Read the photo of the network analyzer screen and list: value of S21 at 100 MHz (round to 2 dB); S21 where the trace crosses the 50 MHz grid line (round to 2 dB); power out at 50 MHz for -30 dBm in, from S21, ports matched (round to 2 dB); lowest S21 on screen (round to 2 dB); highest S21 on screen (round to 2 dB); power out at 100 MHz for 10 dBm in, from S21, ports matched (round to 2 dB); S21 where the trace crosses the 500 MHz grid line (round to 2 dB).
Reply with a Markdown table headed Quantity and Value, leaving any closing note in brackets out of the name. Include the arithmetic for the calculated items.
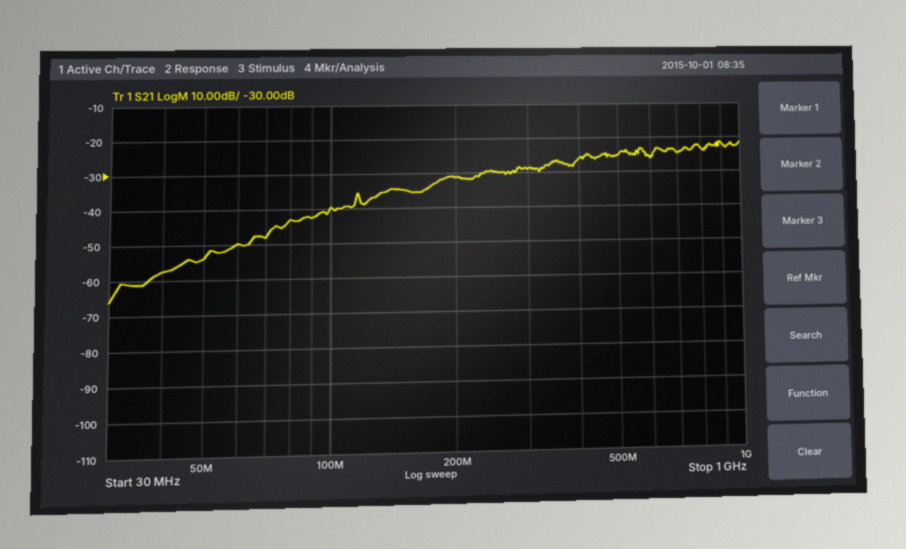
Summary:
| Quantity | Value |
|---|---|
| value of S21 at 100 MHz | -40 dB |
| S21 where the trace crosses the 50 MHz grid line | -54 dB |
| power out at 50 MHz for -30 dBm in, from S21, ports matched | -30 dBm + (-54 dB) = -84 dBm |
| lowest S21 on screen | -66 dB |
| highest S21 on screen | -22 dB |
| power out at 100 MHz for 10 dBm in, from S21, ports matched | 10 dBm + (-40 dB) = -30 dBm |
| S21 where the trace crosses the 500 MHz grid line | -26 dB |
